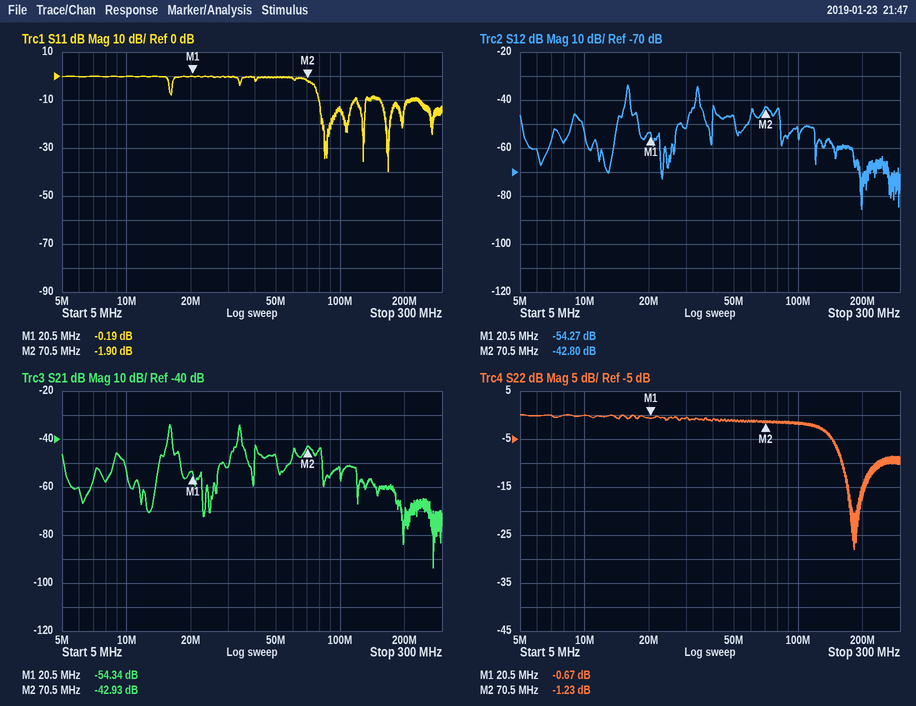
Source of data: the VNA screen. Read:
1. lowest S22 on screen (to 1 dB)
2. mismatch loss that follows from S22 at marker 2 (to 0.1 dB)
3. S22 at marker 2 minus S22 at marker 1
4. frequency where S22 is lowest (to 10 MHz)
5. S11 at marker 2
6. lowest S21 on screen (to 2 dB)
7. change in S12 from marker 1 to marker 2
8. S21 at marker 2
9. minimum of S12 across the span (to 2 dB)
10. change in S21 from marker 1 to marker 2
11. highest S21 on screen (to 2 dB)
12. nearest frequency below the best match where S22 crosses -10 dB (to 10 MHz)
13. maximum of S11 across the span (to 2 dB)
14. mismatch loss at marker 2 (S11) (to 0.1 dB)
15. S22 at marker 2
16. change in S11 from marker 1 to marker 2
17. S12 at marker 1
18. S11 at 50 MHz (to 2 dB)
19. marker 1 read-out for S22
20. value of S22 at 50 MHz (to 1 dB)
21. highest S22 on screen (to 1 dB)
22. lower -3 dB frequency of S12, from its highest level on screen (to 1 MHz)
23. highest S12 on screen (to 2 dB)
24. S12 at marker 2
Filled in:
-28 dB
6.1 dB
-0.56 dB
180 MHz
-1.90 dB
-94 dB
11.47 dB
-42.93 dB
-86 dB
11.41 dB
-34 dB
160 MHz
0 dB
4.5 dB
-1.23 dB
-1.71 dB
-54.27 dB
0 dB
-0.67 dB
-1 dB
0 dB
16 MHz
-34 dB
-42.80 dB
